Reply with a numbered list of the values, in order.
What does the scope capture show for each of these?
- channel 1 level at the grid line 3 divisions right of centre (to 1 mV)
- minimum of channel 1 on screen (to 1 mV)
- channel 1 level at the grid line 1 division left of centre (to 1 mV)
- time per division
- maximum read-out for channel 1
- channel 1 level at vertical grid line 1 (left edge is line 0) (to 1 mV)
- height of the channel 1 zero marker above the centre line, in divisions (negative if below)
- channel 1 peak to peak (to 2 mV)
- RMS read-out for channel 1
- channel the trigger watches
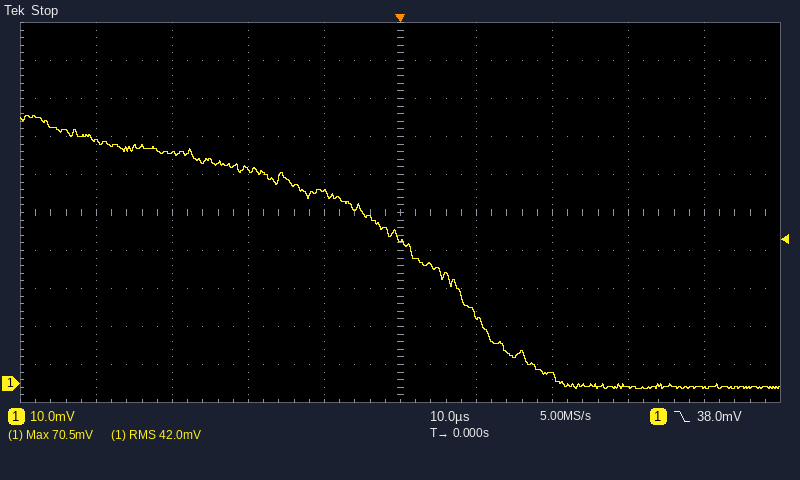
1. -1 mV
2. -1 mV
3. 50 mV
4. 10 µs
5. 70.5 mV
6. 64 mV
7. -4.5 div
8. 72 mV
9. 42.0 mV
10. channel 1
